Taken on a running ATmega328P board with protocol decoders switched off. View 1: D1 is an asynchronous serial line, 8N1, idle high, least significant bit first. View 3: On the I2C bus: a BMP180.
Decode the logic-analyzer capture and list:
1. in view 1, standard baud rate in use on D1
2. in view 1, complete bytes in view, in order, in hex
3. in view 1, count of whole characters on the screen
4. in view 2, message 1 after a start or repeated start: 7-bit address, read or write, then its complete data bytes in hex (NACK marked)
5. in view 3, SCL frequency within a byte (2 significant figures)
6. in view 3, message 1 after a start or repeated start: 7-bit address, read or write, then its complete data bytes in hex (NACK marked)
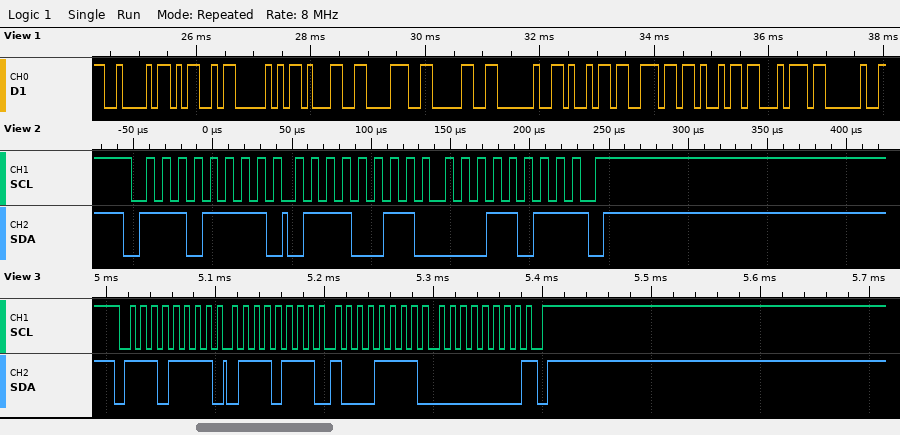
9600 baud
0x42 0x4D 0x50 0x31 0x38 0x30 0x20 0x69 0x6E 0x69 0x74 0x20
12
0x77 read: 73 1B NACK
100 kHz
0x77 read: 77 8F 00 NACK
